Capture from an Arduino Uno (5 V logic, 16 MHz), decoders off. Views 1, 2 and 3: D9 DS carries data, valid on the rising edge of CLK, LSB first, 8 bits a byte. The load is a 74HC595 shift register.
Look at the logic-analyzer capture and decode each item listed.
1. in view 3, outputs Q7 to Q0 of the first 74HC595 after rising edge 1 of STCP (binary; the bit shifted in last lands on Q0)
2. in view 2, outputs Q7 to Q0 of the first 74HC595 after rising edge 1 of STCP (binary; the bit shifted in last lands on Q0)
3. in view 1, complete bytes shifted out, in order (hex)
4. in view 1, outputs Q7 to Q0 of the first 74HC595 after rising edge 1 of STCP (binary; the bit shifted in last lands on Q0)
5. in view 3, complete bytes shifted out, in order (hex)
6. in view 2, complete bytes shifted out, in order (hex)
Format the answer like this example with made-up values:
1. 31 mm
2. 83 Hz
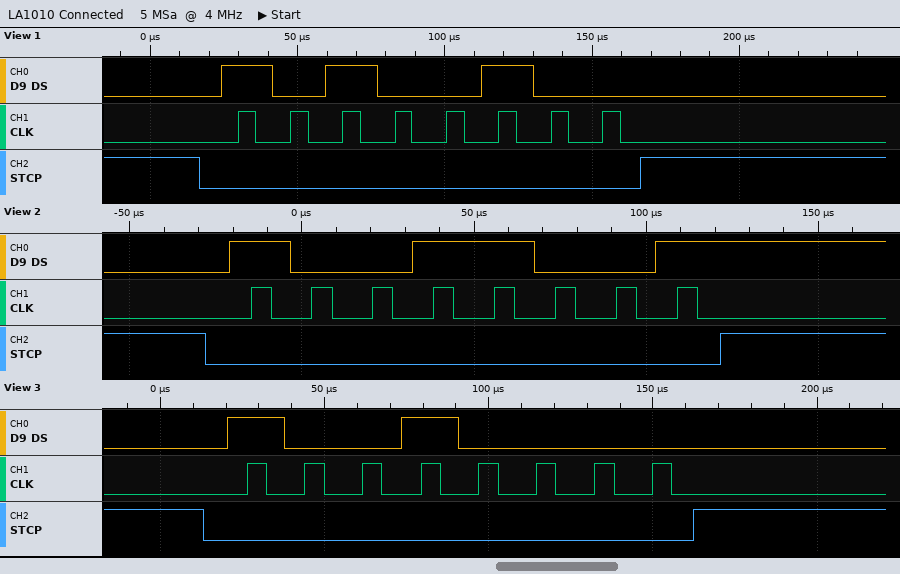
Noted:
1. 10010000
2. 10011001
3. 25
4. 10100100
5. 09
6. 99
